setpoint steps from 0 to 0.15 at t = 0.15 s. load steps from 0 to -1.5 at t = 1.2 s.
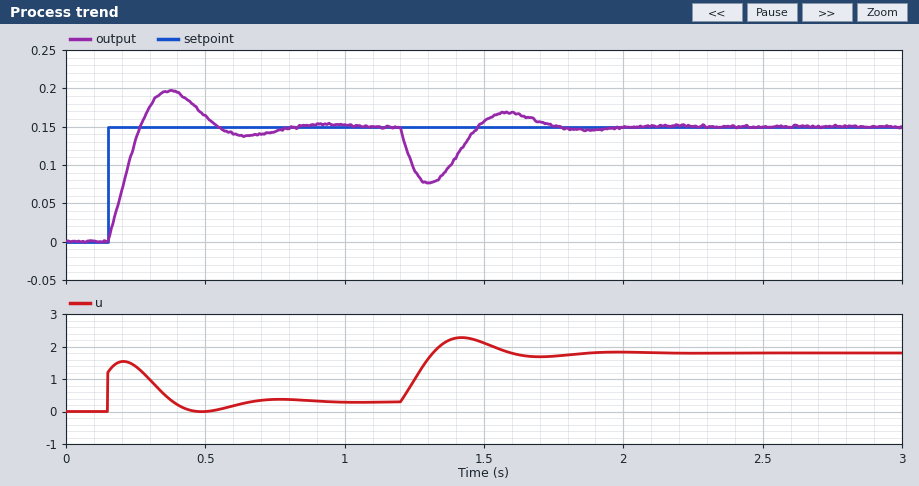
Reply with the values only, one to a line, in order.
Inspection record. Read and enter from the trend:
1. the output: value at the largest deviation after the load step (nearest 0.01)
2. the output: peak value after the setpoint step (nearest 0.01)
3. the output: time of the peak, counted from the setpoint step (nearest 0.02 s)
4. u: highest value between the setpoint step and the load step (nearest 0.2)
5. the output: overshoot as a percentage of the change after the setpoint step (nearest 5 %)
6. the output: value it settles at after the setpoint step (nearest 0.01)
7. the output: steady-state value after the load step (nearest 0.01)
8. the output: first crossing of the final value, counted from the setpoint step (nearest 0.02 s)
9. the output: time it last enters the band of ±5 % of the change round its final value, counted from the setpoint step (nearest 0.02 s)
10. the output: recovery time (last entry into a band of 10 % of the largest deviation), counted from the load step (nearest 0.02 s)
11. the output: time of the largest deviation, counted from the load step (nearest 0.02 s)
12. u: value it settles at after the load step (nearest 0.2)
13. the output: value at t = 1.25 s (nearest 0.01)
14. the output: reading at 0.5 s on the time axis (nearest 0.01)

0.08
0.20
0.22 s
1.6
30 %
0.15
0.15
0.12 s
0.58 s
0.50 s
0.10 s
1.8
0.09
0.16
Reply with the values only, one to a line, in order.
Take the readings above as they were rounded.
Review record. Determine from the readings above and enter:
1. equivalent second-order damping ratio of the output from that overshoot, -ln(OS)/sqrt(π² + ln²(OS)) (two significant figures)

0.36
